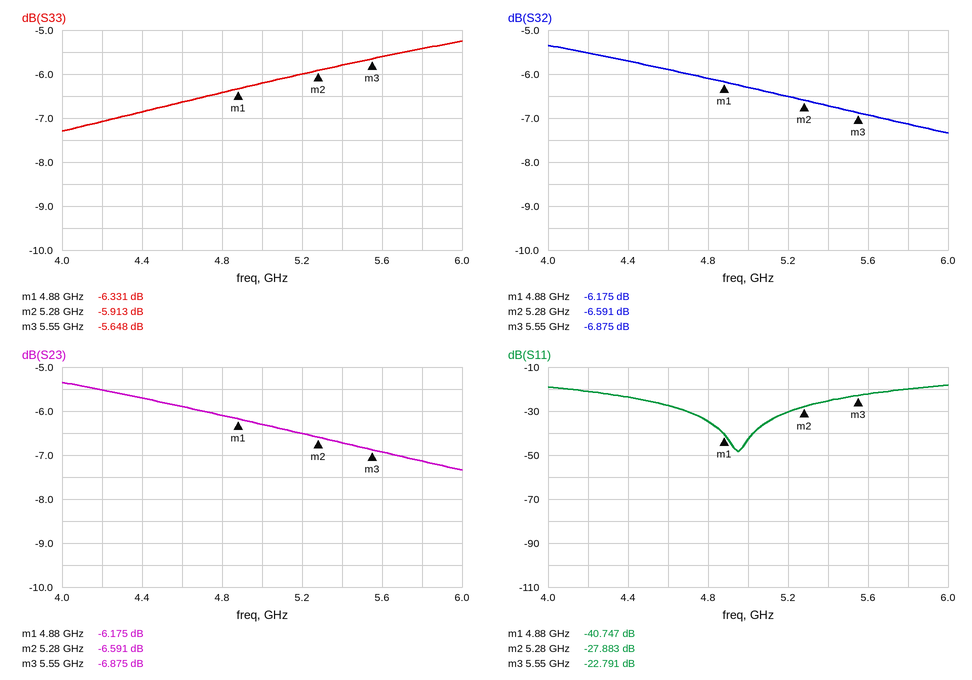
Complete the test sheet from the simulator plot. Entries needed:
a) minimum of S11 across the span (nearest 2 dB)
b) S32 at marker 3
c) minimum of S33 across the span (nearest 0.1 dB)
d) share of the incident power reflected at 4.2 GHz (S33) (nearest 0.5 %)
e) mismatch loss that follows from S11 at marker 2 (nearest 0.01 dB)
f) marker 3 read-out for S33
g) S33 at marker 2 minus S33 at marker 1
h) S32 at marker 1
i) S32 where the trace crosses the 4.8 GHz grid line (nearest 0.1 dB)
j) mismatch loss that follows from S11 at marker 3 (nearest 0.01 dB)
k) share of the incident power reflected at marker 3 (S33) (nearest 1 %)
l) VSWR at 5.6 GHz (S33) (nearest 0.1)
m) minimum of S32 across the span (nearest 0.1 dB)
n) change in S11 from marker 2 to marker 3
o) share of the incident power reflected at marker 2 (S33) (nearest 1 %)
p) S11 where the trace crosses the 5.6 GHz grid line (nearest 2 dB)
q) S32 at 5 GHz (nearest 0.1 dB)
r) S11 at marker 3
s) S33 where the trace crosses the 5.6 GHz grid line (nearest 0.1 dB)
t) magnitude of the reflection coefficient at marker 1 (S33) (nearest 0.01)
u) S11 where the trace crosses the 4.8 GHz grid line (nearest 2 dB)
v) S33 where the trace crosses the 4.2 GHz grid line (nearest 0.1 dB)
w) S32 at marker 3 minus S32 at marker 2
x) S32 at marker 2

-48 dB
-6.875 dB
-7.3 dB
19.5 %
0.01 dB
-5.648 dB
0.418 dB
-6.175 dB
-6.1 dB
0.02 dB
27 %
3.2
-7.3 dB
5.092 dB
26 %
-22 dB
-6.3 dB
-22.791 dB
-5.6 dB
0.48
-34 dB
-7.1 dB
-0.284 dB
-6.591 dB
